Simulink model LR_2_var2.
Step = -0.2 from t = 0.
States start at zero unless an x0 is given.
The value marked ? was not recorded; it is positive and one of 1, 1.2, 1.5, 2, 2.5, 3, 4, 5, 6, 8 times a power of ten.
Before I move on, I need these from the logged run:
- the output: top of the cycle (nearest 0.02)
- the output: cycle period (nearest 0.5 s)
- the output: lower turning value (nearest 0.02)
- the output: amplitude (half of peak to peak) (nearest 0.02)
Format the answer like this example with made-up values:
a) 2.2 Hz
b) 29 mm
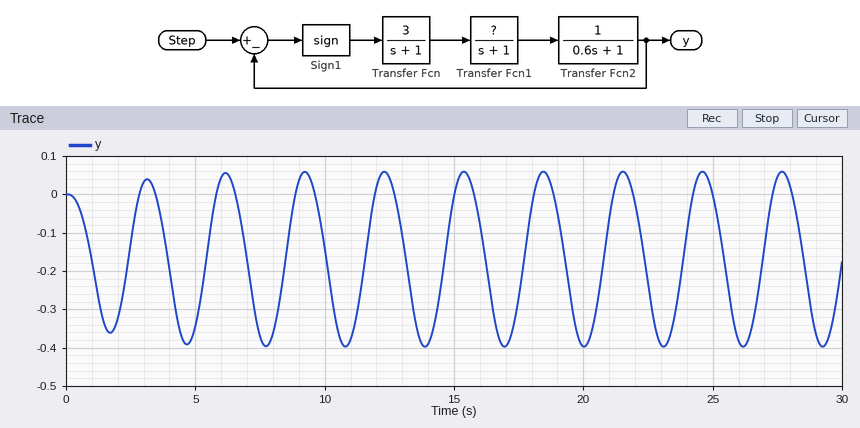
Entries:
a) 0.06
b) 3.0 s
c) -0.40
d) 0.22
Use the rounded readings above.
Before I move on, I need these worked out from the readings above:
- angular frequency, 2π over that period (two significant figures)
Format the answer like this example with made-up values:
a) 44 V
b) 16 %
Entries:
a) 2.1 rad/s
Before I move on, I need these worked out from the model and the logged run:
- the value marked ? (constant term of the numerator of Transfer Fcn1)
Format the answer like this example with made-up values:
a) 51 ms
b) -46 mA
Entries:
a) 0.5
